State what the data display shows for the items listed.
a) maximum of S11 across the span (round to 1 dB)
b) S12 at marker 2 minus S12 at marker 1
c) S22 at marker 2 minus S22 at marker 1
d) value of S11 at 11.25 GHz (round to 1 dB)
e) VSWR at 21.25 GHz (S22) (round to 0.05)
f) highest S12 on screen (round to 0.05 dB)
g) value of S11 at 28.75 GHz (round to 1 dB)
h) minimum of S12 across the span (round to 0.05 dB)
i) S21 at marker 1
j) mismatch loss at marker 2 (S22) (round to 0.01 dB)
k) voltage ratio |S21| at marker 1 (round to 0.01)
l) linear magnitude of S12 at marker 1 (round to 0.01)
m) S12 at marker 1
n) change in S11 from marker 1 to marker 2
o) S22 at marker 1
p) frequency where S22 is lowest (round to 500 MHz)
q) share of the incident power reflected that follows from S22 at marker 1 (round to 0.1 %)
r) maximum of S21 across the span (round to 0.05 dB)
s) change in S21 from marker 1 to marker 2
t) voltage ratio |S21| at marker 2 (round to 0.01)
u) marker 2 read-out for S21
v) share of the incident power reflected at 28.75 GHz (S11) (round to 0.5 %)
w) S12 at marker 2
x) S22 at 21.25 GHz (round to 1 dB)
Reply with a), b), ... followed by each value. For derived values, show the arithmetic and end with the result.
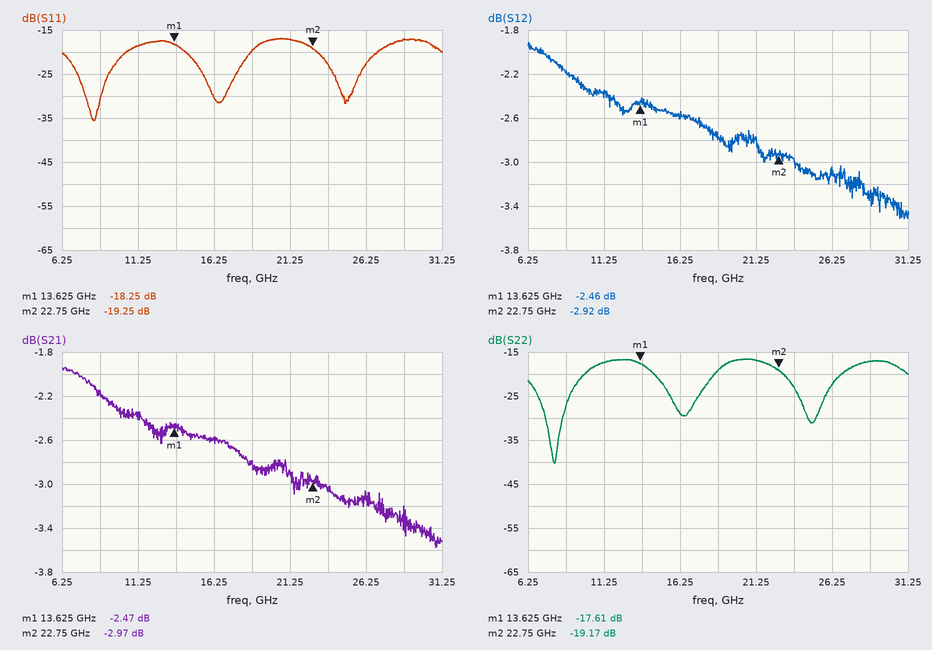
a) -17 dB
b) -2.92 − (-2.46) = -0.46 dB
c) -19.17 − (-17.61) = -1.56 dB
d) -19 dB
e) |Γ| = 10^(-17/20) = 0.1413; VSWR = (1 + 0.1413)/(1 − 0.1413) ≈ 1.33, so 1.35 to the nearest 0.05
f) -1.90 dB
g) -17 dB
h) -3.50 dB
i) -2.47 dB
j) −10 log10(1 − 10^(-19.17/10)) ≈ 0.05 dB
k) 10^(-2.47/20) ≈ 0.75
l) 10^(-2.46/20) ≈ 0.75
m) -2.46 dB
n) -19.25 − (-18.25) = -1.00 dB
o) -17.61 dB
p) 8.0 GHz
q) 10^(-17.61/10) ≈ 1.7 %
r) -1.95 dB
s) -2.97 − (-2.47) = -0.50 dB
t) 10^(-2.97/20) ≈ 0.71
u) -2.97 dB
v) 10^(-17/10) ≈ 2.0 %
w) -2.92 dB
x) -17 dB
